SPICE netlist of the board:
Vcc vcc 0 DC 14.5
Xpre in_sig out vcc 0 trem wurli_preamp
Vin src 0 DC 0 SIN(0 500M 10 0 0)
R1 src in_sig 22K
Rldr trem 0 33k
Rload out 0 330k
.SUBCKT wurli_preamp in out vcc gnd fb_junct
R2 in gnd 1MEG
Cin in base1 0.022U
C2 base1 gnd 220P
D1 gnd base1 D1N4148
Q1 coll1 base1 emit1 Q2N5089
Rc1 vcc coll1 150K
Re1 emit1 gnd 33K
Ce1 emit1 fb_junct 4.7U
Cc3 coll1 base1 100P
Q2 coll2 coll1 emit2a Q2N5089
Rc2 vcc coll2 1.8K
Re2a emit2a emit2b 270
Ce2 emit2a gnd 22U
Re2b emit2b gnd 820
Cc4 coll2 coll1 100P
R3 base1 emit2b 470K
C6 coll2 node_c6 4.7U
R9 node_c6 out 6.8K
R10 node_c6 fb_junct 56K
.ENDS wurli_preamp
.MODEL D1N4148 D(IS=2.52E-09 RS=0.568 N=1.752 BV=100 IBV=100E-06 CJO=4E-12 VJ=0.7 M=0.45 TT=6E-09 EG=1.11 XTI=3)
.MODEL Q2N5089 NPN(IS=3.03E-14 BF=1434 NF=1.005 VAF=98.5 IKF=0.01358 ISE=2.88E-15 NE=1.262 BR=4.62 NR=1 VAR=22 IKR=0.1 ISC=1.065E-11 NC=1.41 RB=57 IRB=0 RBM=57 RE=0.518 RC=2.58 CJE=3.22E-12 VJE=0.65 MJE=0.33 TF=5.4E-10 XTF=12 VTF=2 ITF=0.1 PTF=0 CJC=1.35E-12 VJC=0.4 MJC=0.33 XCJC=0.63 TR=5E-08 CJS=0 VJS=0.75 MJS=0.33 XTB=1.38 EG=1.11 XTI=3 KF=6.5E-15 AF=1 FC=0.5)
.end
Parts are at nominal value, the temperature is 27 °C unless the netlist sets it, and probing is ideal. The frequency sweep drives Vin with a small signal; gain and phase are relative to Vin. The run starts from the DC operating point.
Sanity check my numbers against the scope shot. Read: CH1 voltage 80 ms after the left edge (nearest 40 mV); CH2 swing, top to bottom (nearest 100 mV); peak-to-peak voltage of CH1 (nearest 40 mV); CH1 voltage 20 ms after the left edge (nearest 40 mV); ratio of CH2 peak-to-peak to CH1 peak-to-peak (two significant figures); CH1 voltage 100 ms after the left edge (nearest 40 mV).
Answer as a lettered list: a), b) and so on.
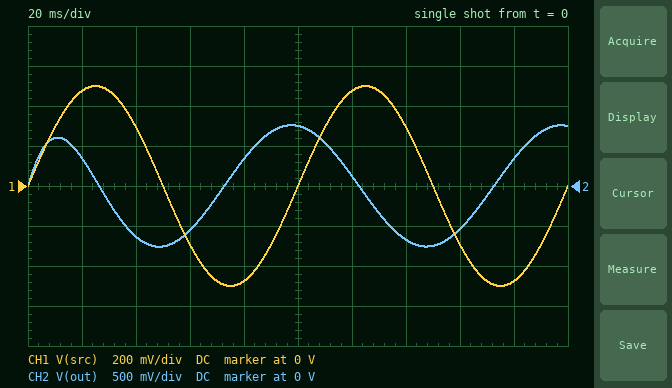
a) -480 mV
b) 1.5 V
c) 1.00 V
d) 480 mV
e) 1.5
f) 0 V
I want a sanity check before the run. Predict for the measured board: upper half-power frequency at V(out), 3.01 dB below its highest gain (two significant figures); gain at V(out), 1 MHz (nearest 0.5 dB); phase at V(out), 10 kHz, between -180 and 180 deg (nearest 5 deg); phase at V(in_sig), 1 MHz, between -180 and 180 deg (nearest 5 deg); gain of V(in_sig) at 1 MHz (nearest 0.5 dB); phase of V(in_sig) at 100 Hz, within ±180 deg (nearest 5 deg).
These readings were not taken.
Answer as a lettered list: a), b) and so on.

a) 16 kHz
b) -33.0 dB
c) -45 deg
d) -90 deg
e) -33.0 dB
f) 0 deg
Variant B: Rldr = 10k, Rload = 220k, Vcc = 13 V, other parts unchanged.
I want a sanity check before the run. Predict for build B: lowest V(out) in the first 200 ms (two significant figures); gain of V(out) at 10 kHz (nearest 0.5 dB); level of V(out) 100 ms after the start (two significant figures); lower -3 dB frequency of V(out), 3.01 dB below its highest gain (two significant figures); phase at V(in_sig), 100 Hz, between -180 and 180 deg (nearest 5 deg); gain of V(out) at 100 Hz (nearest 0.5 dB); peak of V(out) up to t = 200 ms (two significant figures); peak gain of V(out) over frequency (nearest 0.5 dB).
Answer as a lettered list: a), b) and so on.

a) -1.1 V
b) 15.5 dB
c) 870 mV
d) 18 Hz
e) 0 deg
f) 17.0 dB
g) 990 mV
h) 18.0 dB
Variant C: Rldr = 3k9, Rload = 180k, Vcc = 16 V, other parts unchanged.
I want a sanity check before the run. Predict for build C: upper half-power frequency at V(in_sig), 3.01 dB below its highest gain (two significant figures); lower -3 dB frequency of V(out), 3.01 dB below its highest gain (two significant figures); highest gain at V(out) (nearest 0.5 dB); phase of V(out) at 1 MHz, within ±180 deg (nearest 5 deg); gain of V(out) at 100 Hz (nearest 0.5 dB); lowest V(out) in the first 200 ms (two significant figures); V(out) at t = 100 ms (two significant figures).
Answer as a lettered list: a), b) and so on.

a) 21 kHz
b) 24 Hz
c) 25.5 dB
d) 115 deg
e) 23.5 dB
f) -1.2 V
g) 790 mV
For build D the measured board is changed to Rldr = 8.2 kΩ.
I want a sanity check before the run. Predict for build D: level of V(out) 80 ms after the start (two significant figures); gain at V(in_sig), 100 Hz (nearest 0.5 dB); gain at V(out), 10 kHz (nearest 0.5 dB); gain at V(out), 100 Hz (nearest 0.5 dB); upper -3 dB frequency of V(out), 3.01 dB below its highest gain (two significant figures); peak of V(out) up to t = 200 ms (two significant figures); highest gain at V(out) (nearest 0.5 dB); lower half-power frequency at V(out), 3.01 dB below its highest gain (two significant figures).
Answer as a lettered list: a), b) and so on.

a) 770 mV
b) -0.5 dB
c) 17.0 dB
d) 18.5 dB
e) 12 kHz
f) 1.1 V
g) 19.5 dB
h) 19 Hz
